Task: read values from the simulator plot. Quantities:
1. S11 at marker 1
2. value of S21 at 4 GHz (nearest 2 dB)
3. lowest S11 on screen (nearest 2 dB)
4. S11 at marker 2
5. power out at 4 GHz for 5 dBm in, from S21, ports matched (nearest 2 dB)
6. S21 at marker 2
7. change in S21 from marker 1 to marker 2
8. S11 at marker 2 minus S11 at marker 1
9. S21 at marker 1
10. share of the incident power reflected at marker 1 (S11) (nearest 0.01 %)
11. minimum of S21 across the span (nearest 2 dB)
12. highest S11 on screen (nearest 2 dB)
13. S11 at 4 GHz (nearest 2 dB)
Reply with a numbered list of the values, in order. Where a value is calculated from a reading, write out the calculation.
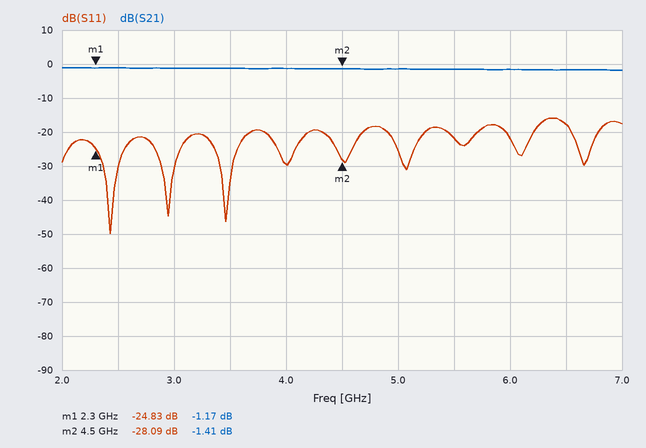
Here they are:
1. -24.83 dB
2. -2 dB
3. -50 dB
4. -28.09 dB
5. 5 dBm + (-2 dB) = 4 dBm
6. -1.41 dB
7. -1.41 − (-1.17) = -0.24 dB
8. -28.09 − (-24.83) = -3.26 dB
9. -1.17 dB
10. 10^(-24.83/10) ≈ 0.33 %
11. -2 dB
12. -16 dB
13. -30 dB
